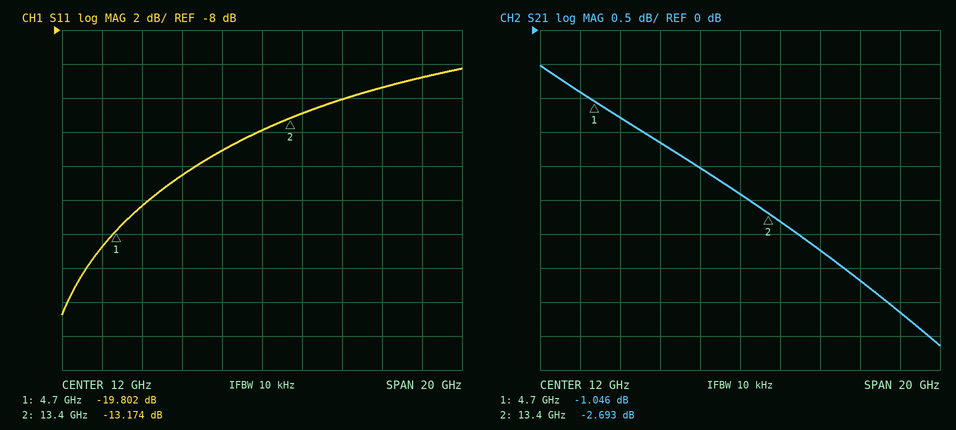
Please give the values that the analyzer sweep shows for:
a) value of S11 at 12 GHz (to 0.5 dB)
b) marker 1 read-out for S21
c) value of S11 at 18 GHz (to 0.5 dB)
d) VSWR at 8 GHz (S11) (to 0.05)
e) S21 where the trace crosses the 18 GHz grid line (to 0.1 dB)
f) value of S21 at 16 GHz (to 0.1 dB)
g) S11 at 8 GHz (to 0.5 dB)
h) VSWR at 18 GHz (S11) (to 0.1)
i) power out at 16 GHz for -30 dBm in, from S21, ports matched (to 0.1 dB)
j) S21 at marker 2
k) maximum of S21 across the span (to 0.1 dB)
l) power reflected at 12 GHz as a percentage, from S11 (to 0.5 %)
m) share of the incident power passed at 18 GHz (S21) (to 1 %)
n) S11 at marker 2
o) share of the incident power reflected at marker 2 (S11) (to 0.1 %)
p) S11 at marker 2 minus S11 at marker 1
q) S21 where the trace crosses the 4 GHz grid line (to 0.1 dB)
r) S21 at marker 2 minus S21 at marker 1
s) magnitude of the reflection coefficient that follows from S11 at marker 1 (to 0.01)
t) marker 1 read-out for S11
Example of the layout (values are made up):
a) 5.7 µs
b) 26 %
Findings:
a) -14.0 dB
b) -1.046 dB
c) -11.5 dB
d) 1.35
e) -3.7 dB
f) -3.2 dB
g) -16.5 dB
h) 1.7
i) -33.2 dBm
j) -2.693 dB
k) -0.5 dB
l) 4.0 %
m) 43 %
n) -13.174 dB
o) 4.8 %
p) 6.628 dB
q) -0.9 dB
r) -1.647 dB
s) 0.10
t) -19.802 dB
